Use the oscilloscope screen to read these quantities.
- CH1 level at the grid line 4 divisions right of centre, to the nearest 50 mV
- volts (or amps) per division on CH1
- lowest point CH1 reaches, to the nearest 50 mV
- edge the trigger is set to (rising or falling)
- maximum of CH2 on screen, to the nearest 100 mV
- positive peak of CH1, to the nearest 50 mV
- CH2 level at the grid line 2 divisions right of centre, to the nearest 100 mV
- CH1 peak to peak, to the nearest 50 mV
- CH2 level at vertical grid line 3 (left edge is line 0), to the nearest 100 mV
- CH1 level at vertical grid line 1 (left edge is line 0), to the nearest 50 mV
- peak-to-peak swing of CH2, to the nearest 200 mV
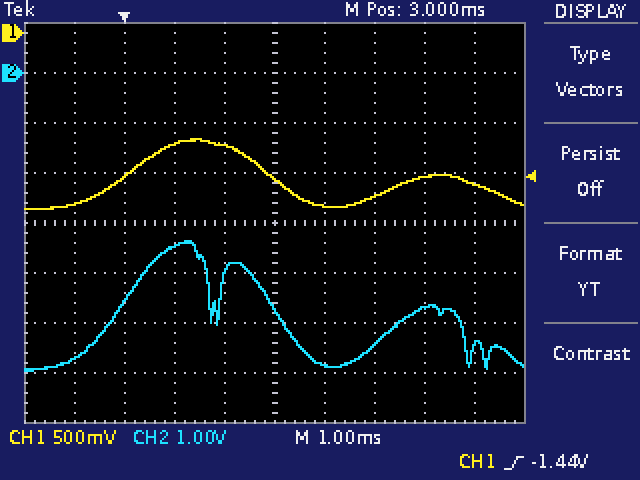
-1.50 V
500 mV
-1.75 V
rising
-3.4 V
-1.05 V
-5.4 V
700 mV
-3.5 V
-1.70 V
2.6 V
